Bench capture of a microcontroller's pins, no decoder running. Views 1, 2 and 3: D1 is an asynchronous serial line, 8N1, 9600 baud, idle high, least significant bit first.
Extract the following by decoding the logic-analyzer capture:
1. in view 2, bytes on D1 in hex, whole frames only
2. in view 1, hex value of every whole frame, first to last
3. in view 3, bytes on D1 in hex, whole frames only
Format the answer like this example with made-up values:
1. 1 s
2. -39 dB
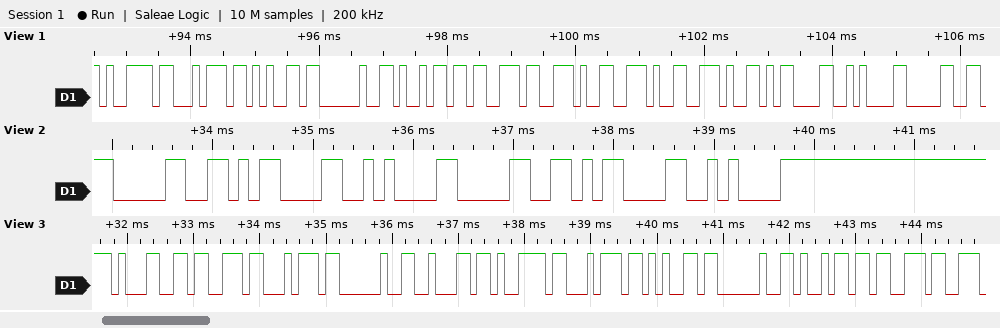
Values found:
1. 30 0D 0A 30 0D 0A
2. 79 74 65 20 69 73 2E 2E 2E 0D 0A 30
3. 31 73 74 20 62 79 74 65 20 69 73
